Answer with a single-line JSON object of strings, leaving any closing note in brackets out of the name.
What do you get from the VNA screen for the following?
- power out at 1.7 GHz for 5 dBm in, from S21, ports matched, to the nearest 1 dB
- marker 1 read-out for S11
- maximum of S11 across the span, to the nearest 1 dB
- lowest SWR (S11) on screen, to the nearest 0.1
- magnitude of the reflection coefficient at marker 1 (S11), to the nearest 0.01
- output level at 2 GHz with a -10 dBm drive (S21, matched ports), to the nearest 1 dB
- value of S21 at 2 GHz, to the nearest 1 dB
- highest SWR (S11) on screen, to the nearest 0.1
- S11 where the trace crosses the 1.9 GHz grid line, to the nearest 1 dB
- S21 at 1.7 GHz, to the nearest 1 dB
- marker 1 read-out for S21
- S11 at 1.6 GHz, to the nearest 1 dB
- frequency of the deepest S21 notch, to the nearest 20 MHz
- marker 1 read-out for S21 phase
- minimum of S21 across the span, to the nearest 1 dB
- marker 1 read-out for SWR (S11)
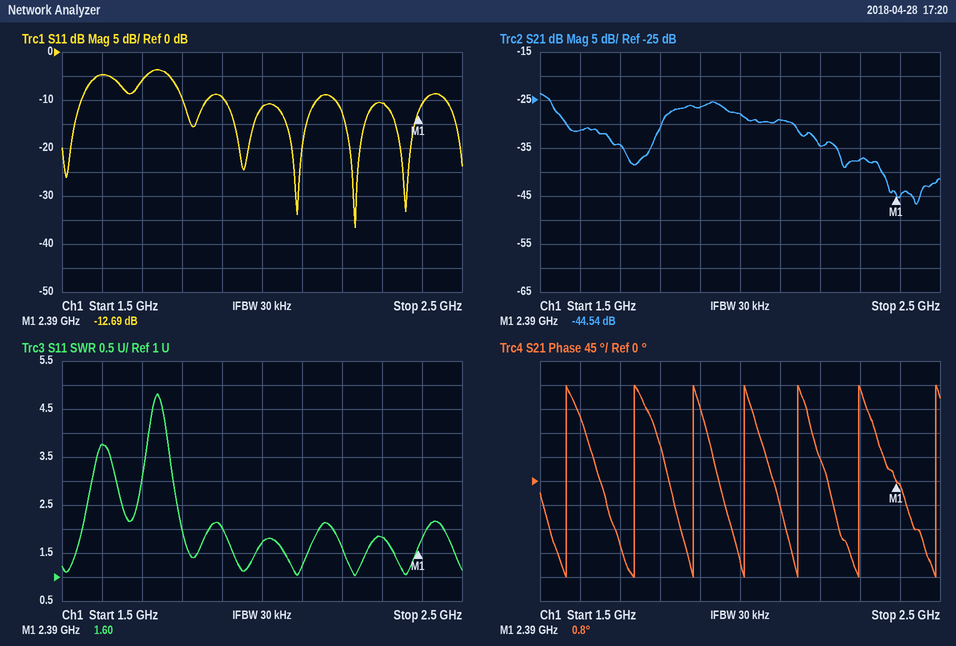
{"power out at 1.7 GHz for 5 dBm in, from S21, ports matched, to the nearest 1 dB": "-29 dBm", "marker 1 read-out for S11": "-12.69 dB", "maximum of S11 across the span, to the nearest 1 dB": "-4 dB", "lowest SWR (S11) on screen, to the nearest 0.1": "1.0", "magnitude of the reflection coefficient at marker 1 (S11), to the nearest 0.01": "0.23", "output level at 2 GHz with a -10 dBm drive (S21, matched ports), to the nearest 1 dB": "-38 dBm", "value of S21 at 2 GHz, to the nearest 1 dB": "-28 dB", "highest SWR (S11) on screen, to the nearest 0.1": "4.8", "S11 where the trace crosses the 1.9 GHz grid line, to the nearest 1 dB": "-9 dB", "S21 at 1.7 GHz, to the nearest 1 dB": "-34 dB", "marker 1 read-out for S21": "-44.54 dB", "S11 at 1.6 GHz, to the nearest 1 dB": "-5 dB", "frequency of the deepest S21 notch, to the nearest 20 MHz": "2.44 GHz", "marker 1 read-out for S21 phase": "0.8°", "minimum of S21 across the span, to the nearest 1 dB": "-47 dB", "marker 1 read-out for SWR": "1.60"}
